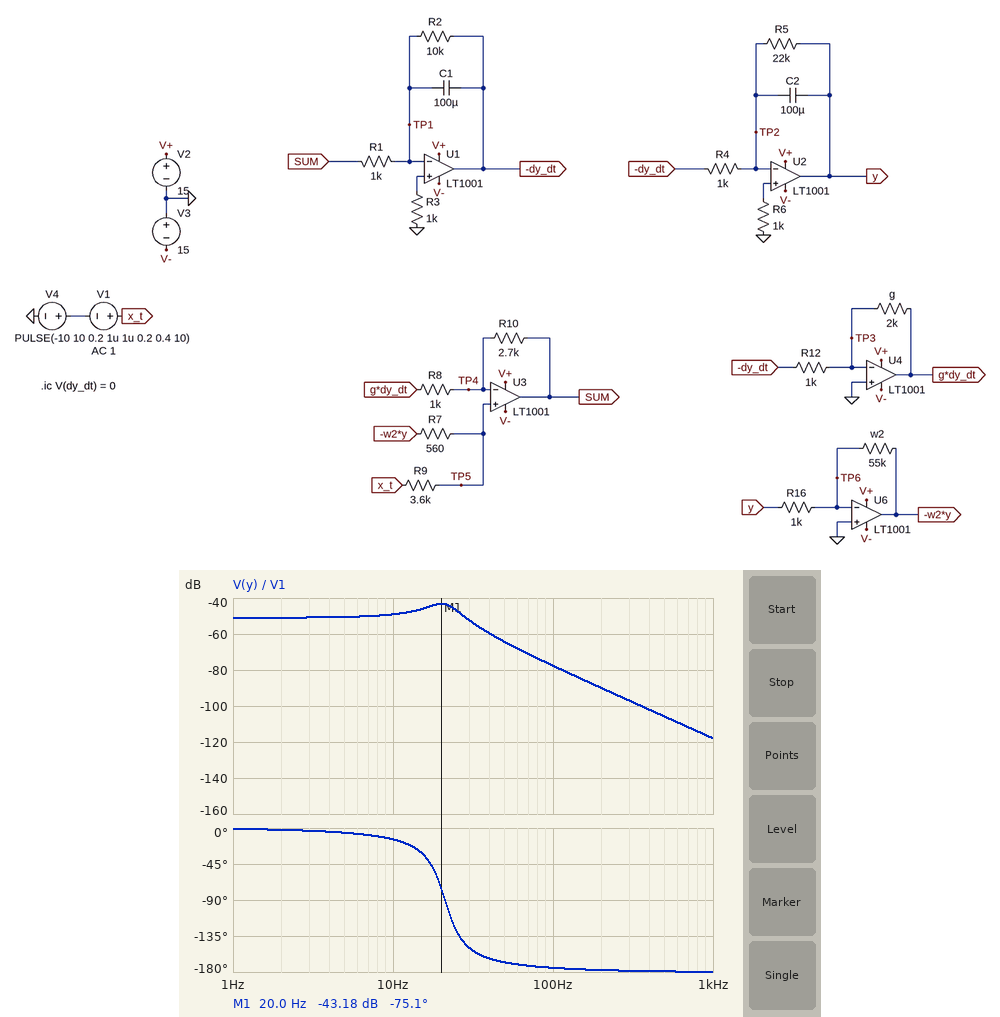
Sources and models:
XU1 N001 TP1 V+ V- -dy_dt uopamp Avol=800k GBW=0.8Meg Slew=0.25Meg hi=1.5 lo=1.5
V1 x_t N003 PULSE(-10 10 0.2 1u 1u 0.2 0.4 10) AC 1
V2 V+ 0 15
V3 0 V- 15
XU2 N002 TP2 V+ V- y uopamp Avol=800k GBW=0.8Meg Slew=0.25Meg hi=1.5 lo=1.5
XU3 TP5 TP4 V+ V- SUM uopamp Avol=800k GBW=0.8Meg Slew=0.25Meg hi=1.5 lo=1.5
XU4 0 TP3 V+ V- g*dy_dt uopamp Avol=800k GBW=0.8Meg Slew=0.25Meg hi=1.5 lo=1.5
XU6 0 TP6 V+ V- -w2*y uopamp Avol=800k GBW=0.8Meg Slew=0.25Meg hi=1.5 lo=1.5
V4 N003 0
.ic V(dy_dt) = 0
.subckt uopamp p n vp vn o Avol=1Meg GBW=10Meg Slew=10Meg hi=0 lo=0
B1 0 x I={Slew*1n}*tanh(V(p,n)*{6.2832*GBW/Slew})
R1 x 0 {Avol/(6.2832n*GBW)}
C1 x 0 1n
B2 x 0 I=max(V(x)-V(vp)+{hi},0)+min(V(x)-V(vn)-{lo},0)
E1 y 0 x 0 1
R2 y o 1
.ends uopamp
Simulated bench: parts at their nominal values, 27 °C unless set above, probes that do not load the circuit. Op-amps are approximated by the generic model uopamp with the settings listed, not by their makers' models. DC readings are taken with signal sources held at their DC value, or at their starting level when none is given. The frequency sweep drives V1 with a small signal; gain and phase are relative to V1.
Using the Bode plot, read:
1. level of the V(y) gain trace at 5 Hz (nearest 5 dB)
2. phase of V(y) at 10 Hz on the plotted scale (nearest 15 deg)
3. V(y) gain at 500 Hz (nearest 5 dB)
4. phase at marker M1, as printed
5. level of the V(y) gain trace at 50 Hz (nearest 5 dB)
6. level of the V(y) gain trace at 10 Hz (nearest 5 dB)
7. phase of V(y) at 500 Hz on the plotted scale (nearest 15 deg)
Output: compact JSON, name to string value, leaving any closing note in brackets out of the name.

{"level of the V(y) gain trace at 5 Hz": "-50 dB", "phase of V(y) at 10 Hz on the plotted scale": "-15 deg", "V(y) gain at 500 Hz": "-105 dB", "phase at marker M1, as printed": "-75.1 deg", "level of the V(y) gain trace at 50 Hz": "-65 dB", "level of the V(y) gain trace at 10 Hz": "-50 dB", "phase of V(y) at 500 Hz on the plotted scale": "-180 deg"}
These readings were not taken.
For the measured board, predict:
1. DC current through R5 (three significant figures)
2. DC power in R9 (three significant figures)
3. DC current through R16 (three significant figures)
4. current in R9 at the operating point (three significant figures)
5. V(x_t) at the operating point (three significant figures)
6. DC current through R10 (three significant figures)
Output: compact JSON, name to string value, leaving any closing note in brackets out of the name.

{"DC current through R5": "1.28 µA", "DC power in R9": "27.8 mW", "DC current through R16": "28.2 µA", "current in R9 at the operating point": "2.78 mA", "V(x_t) at the operating point": "-10.0 V", "DC current through R10": "659 nA"}
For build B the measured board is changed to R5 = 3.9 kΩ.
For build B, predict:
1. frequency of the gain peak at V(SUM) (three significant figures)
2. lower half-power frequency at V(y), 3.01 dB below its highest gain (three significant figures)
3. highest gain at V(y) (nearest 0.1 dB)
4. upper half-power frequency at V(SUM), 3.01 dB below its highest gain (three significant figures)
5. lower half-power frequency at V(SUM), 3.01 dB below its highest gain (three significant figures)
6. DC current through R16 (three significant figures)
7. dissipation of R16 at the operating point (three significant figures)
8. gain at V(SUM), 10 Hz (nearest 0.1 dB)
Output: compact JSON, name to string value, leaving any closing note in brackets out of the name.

{"frequency of the gain peak at V(SUM)": "22.3 Hz", "lower half-power frequency at V(y), 3.01 dB below its highest gain": "14.8 Hz", "highest gain at V(y)": "-43.5 dB", "upper half-power frequency at V(SUM), 3.01 dB below its highest gain": "30.4 Hz", "lower half-power frequency at V(SUM), 3.01 dB below its highest gain": "18.4 Hz", "DC current through R16": "28.1 µA", "dissipation of R16 at the operating point": "787 nW", "gain at V(SUM), 10 Hz": "-17.2 dB"}
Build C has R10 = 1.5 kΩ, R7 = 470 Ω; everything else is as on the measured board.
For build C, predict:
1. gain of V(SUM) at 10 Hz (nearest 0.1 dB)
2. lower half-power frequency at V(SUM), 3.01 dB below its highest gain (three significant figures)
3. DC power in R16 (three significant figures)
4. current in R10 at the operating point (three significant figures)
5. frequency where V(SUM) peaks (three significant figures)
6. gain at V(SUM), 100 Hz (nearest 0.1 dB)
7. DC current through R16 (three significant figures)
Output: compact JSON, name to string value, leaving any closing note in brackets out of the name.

{"gain of V(SUM) at 10 Hz": "-17.4 dB", "lower half-power frequency at V(SUM), 3.01 dB below its highest gain": "15.8 Hz", "DC power in R16": "562 nW", "current in R10 at the operating point": "819 nA", "frequency where V(SUM) peaks": "17.9 Hz", "gain at V(SUM), 100 Hz": "-10.5 dB", "DC current through R16": "23.7 µA"}
